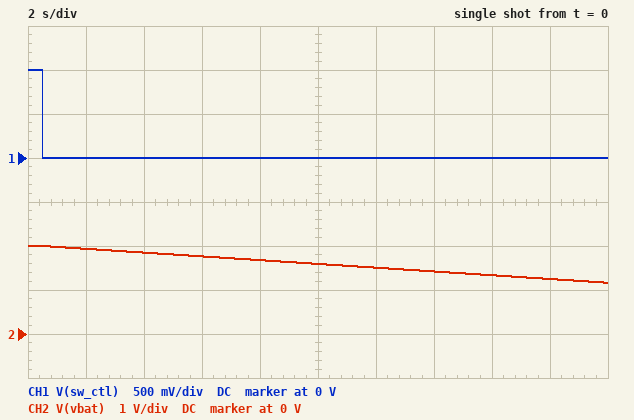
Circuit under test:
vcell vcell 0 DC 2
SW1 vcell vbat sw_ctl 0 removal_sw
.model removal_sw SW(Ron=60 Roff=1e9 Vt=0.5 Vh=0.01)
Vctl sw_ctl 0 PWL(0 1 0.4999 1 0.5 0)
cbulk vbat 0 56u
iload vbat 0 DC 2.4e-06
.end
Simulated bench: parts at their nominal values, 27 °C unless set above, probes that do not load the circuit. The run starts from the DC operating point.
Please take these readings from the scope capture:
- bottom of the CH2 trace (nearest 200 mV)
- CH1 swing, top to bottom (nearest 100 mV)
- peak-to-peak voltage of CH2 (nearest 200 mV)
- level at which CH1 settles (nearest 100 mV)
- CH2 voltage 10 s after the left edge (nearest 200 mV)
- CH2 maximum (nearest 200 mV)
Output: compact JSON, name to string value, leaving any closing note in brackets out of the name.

{"bottom of the CH2 trace": "1.2 V", "CH1 swing, top to bottom": "1.0 V", "peak-to-peak voltage of CH2": "800 mV", "level at which CH1 settles": "0 V", "CH2 voltage 10 s after the left edge": "1.6 V", "CH2 maximum": "2.0 V"}
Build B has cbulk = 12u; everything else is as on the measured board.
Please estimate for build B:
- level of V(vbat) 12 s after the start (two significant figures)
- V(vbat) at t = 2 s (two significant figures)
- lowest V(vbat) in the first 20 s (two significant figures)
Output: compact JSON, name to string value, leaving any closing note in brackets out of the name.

{"level of V(vbat) 12 s after the start": "-300 mV", "V(vbat) at t = 2 s": "1.7 V", "lowest V(vbat) in the first 20 s": "-1.9 V"}
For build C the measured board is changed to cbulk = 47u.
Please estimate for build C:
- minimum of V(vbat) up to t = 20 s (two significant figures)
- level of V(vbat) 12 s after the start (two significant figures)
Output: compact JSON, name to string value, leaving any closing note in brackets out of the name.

{"minimum of V(vbat) up to t = 20 s": "1.0 V", "level of V(vbat) 12 s after the start": "1.4 V"}
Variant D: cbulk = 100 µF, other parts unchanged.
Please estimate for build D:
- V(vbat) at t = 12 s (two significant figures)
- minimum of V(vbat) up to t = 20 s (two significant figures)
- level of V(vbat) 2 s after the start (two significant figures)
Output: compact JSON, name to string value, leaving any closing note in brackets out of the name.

{"V(vbat) at t = 12 s": "1.7 V", "minimum of V(vbat) up to t = 20 s": "1.5 V", "level of V(vbat) 2 s after the start": "2.0 V"}
